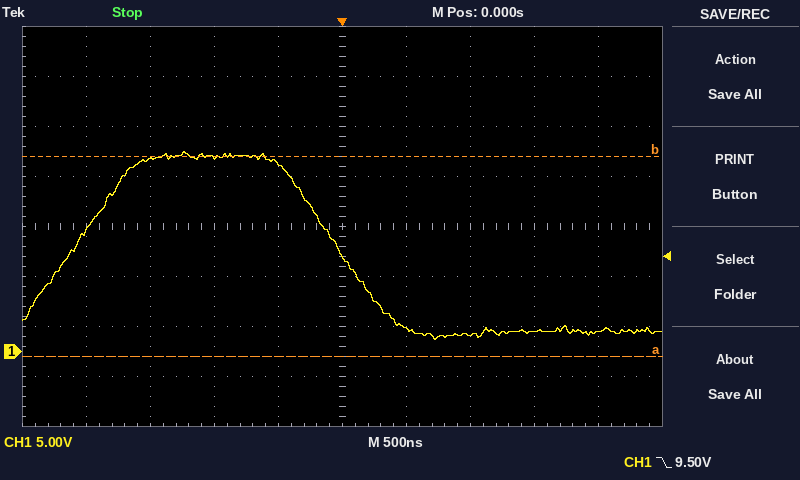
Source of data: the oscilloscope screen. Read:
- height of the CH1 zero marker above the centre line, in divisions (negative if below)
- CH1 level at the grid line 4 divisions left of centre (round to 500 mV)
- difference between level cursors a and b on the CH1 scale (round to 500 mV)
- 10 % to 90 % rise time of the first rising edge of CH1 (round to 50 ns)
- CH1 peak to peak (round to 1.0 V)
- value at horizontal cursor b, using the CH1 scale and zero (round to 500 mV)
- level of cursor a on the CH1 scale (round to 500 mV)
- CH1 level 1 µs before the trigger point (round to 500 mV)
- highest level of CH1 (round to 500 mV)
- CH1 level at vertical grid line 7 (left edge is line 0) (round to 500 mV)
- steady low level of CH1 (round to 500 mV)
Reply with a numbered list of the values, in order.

1. -2.5 div
2. 12.0 V
3. 20.0 V
4. 750 ns
5. 19.0 V
6. 19.5 V
7. -500 mV
8. 19.5 V
9. 20.0 V
10. 1.5 V
11. 2.0 V
